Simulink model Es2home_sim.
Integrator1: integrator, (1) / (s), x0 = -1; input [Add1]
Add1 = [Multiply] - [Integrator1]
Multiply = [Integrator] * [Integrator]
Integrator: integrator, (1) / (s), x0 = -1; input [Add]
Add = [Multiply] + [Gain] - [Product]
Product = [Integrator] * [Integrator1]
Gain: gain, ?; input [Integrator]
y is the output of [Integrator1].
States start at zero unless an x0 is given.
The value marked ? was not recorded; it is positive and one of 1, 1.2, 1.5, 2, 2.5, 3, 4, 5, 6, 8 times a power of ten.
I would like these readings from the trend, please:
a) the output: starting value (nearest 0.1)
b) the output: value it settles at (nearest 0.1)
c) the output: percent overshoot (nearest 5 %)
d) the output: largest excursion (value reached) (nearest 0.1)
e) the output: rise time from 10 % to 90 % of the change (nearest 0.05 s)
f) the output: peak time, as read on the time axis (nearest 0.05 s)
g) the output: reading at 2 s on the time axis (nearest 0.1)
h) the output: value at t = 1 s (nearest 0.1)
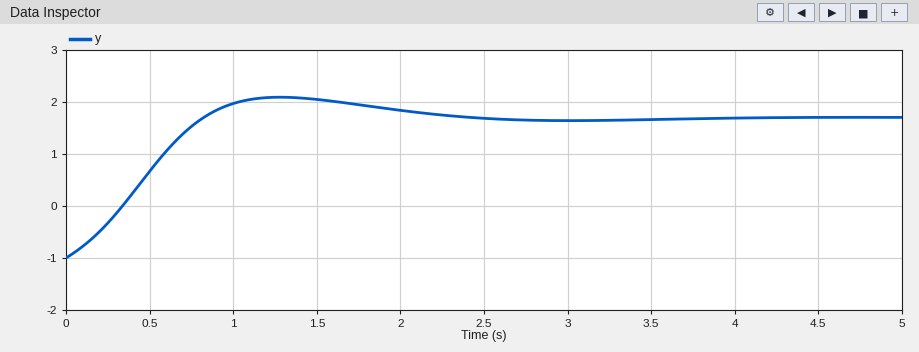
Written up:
-1.0
1.7
15 %
2.1
0.60 s
1.30 s
1.8
2.0
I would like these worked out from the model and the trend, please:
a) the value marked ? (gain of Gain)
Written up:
3
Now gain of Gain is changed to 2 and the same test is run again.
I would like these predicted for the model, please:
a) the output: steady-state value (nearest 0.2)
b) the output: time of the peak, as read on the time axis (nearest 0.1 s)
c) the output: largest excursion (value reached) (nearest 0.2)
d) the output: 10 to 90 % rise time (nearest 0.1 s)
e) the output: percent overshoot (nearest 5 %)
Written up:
1.0
1.5 s
1.2
0.7 s
15 %
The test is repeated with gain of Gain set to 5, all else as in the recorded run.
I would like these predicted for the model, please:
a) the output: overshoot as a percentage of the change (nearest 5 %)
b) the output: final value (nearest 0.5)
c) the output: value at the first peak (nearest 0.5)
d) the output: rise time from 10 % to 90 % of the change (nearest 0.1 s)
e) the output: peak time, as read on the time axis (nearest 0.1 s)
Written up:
15 %
3.0
4.0
0.4 s
1.0 s
